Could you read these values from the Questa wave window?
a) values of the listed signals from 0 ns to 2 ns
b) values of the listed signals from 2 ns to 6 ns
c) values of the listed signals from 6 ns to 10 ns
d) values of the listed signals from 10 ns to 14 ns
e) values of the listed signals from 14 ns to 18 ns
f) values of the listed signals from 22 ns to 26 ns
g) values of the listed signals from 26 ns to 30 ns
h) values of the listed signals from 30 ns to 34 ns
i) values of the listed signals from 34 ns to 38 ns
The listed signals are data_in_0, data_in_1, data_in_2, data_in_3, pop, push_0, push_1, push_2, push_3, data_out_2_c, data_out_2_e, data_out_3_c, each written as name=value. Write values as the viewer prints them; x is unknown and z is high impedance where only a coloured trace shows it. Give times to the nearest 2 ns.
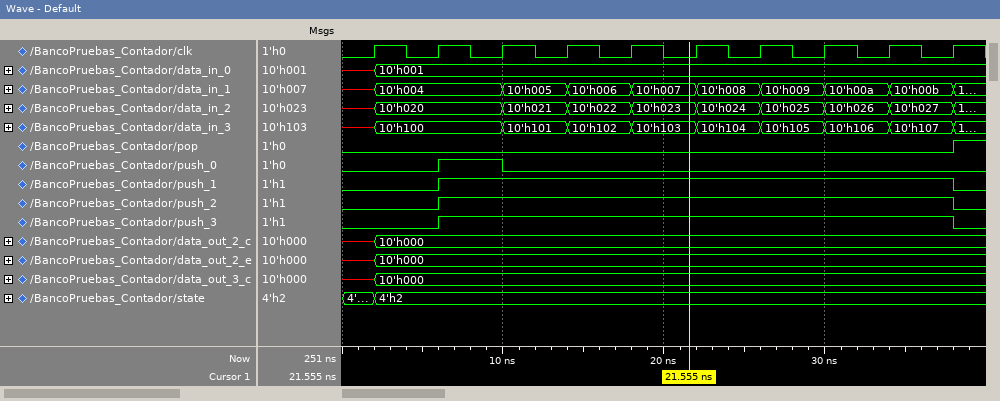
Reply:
data_in_0=x, data_in_1=x, data_in_2=x, data_in_3=x, pop=0, push_0=0, push_1=0, push_2=0, push_3=0, data_out_2_c=x, data_out_2_e=x, data_out_3_c=x
data_in_0=10'h001, data_in_1=10'h004, data_in_2=10'h020, data_in_3=10'h100, pop=0, push_0=0, push_1=0, push_2=0, push_3=0, data_out_2_c=10'h000, data_out_2_e=10'h000, data_out_3_c=10'h000
data_in_0=10'h001, data_in_1=10'h004, data_in_2=10'h020, data_in_3=10'h100, pop=0, push_0=1, push_1=1, push_2=1, push_3=1, data_out_2_c=10'h000, data_out_2_e=10'h000, data_out_3_c=10'h000
data_in_0=10'h001, data_in_1=10'h005, data_in_2=10'h021, data_in_3=10'h101, pop=0, push_0=0, push_1=1, push_2=1, push_3=1, data_out_2_c=10'h000, data_out_2_e=10'h000, data_out_3_c=10'h000
data_in_0=10'h001, data_in_1=10'h006, data_in_2=10'h022, data_in_3=10'h102, pop=0, push_0=0, push_1=1, push_2=1, push_3=1, data_out_2_c=10'h000, data_out_2_e=10'h000, data_out_3_c=10'h000
data_in_0=10'h001, data_in_1=10'h008, data_in_2=10'h024, data_in_3=10'h104, pop=0, push_0=0, push_1=1, push_2=1, push_3=1, data_out_2_c=10'h000, data_out_2_e=10'h000, data_out_3_c=10'h000
data_in_0=10'h001, data_in_1=10'h009, data_in_2=10'h025, data_in_3=10'h105, pop=0, push_0=0, push_1=1, push_2=1, push_3=1, data_out_2_c=10'h000, data_out_2_e=10'h000, data_out_3_c=10'h000
data_in_0=10'h001, data_in_1=10'h00a, data_in_2=10'h026, data_in_3=10'h106, pop=0, push_0=0, push_1=1, push_2=1, push_3=1, data_out_2_c=10'h000, data_out_2_e=10'h000, data_out_3_c=10'h000
data_in_0=10'h001, data_in_1=10'h00b, data_in_2=10'h027, data_in_3=10'h107, pop=0, push_0=0, push_1=1, push_2=1, push_3=1, data_out_2_c=10'h000, data_out_2_e=10'h000, data_out_3_c=10'h000
